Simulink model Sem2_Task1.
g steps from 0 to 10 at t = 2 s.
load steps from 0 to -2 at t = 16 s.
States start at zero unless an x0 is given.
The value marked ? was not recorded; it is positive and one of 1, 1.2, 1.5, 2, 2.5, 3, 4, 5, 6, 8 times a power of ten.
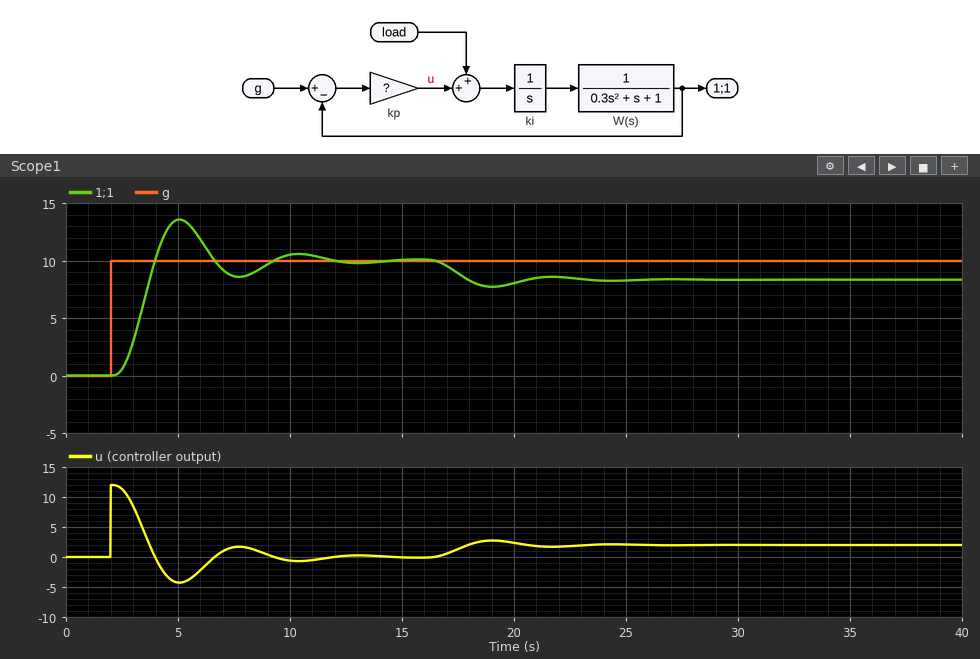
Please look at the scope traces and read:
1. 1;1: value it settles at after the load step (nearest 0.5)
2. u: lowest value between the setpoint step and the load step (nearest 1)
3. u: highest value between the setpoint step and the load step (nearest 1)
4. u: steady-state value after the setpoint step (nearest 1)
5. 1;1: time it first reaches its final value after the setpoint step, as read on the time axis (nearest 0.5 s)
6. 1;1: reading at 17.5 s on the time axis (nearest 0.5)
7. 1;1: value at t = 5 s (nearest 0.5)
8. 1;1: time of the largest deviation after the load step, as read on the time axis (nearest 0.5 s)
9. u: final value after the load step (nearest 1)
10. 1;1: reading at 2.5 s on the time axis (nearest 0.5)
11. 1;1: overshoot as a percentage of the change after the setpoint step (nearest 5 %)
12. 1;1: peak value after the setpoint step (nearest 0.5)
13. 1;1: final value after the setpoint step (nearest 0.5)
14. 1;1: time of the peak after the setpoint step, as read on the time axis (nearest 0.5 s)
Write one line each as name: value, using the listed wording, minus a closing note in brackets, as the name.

1;1: value it settles at after the load step: 8.5
u: lowest value between the setpoint step and the load step: -4
u: highest value between the setpoint step and the load step: 12
u: steady-state value after the setpoint step: 0
1;1: time it first reaches its final value after the setpoint step, as read on the time axis: 4.0 s
1;1: reading at 17.5 s on the time axis: 9.0
1;1: value at t = 5 s: 13.5
1;1: time of the largest deviation after the load step, as read on the time axis: 19.0 s
u: final value after the load step: 2
1;1: reading at 2.5 s on the time axis: 0.5
1;1: overshoot as a percentage of the change after the setpoint step: 35 %
1;1: peak value after the setpoint step: 13.5
1;1: final value after the setpoint step: 10.0
1;1: time of the peak after the setpoint step, as read on the time axis: 5.0 s
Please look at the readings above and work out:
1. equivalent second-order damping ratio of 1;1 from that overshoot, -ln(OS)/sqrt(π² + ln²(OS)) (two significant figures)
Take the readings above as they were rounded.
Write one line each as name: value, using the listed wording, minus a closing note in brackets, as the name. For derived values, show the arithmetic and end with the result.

equivalent second-order damping ratio of 1;1 from that overshoot, -ln(OS)/sqrt(π² + ln²(OS)): ln(0.35) = -1.050; 1.050 / sqrt(9.870 + 1.102) = 0.32
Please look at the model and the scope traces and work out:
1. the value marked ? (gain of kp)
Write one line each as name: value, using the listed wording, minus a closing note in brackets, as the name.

the value marked ?: 1.2
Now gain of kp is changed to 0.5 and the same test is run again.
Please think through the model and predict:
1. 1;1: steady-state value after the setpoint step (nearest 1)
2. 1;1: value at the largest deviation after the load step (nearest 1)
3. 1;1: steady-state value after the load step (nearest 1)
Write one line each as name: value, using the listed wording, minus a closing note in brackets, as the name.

1;1: steady-state value after the setpoint step: 10
1;1: value at the largest deviation after the load step: 6
1;1: steady-state value after the load step: 6
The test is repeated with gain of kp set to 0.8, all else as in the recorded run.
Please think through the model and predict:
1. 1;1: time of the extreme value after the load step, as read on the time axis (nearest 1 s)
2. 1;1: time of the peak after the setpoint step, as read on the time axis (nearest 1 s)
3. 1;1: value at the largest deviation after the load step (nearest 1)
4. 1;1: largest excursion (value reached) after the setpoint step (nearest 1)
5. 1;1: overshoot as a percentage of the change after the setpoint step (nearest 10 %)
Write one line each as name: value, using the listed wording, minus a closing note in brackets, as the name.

1;1: time of the extreme value after the load step, as read on the time axis: 20 s
1;1: time of the peak after the setpoint step, as read on the time axis: 6 s
1;1: value at the largest deviation after the load step: 7
1;1: largest excursion (value reached) after the setpoint step: 12
1;1: overshoot as a percentage of the change after the setpoint step: 20 %
